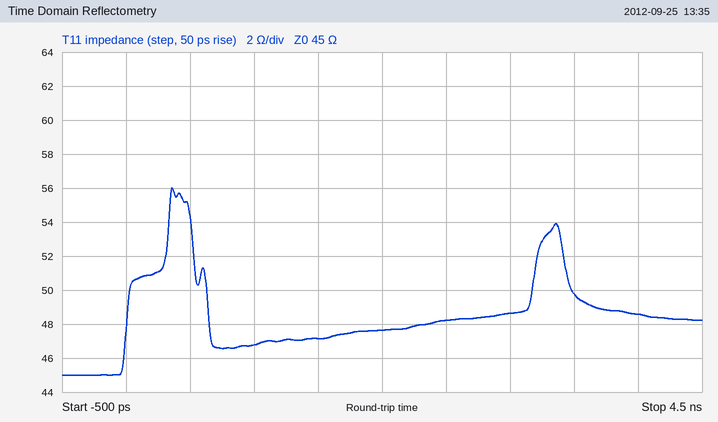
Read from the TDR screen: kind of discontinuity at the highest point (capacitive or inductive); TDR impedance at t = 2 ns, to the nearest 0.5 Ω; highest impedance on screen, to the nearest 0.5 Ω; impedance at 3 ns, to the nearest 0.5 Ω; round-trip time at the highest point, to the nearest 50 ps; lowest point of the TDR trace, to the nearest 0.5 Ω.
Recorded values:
inductive
47.5 Ω
56.0 Ω
48.5 Ω
350 ps
45.0 Ω
